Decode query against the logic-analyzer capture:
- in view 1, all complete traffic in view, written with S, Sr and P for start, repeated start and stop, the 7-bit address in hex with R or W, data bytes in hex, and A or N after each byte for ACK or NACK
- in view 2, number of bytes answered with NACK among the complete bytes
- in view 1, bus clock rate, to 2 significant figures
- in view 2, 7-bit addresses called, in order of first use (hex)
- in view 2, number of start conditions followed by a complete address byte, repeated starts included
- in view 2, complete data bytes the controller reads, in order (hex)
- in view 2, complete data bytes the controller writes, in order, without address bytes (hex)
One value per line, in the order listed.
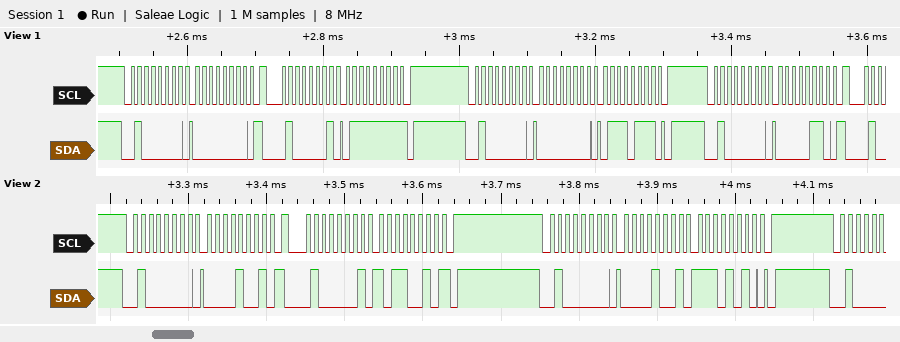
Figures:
S 20W A 00 A Sr 20R A 7F N P S 20W A 00 A 77 A P S 20W A 06 A
1
100 kHz
0x20
3
B2
09 09 EA
